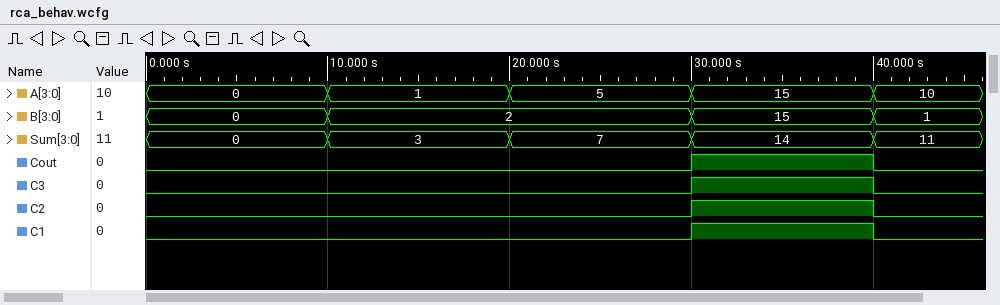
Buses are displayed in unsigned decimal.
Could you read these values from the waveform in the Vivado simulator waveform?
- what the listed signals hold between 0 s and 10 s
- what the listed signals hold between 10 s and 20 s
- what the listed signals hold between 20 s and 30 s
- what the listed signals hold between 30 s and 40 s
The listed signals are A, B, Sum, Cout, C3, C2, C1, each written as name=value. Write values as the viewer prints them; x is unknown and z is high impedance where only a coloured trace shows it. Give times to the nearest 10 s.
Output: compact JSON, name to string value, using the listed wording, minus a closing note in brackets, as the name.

{"what the listed signals hold between 0 s and 10 s": "A=0, B=0, Sum=0, Cout=0, C3=0, C2=0, C1=0", "what the listed signals hold between 10 s and 20 s": "A=1, B=2, Sum=3, Cout=0, C3=0, C2=0, C1=0", "what the listed signals hold between 20 s and 30 s": "A=5, B=2, Sum=7, Cout=0, C3=0, C2=0, C1=0", "what the listed signals hold between 30 s and 40 s": "A=15, B=15, Sum=14, Cout=1, C3=1, C2=1, C1=1"}
